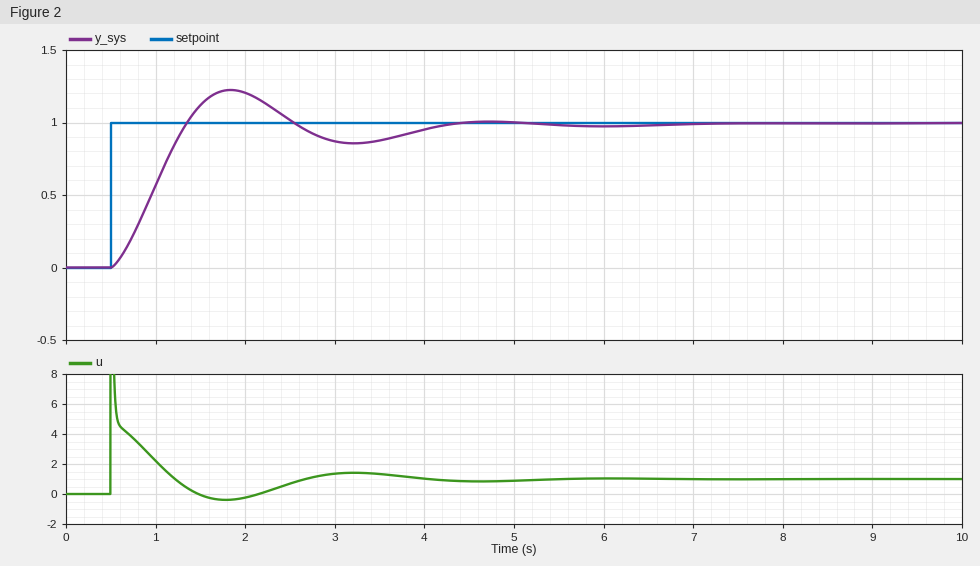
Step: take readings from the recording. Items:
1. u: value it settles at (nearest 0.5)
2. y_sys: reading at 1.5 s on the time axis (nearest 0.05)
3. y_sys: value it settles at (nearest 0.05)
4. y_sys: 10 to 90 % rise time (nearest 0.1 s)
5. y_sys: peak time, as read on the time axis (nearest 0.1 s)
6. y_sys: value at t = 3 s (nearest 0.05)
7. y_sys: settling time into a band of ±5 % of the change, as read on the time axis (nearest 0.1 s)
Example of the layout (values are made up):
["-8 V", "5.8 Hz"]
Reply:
["1.0", "1.10", "1.00", "0.6 s", "1.8 s", "0.85", "4.0 s"]
